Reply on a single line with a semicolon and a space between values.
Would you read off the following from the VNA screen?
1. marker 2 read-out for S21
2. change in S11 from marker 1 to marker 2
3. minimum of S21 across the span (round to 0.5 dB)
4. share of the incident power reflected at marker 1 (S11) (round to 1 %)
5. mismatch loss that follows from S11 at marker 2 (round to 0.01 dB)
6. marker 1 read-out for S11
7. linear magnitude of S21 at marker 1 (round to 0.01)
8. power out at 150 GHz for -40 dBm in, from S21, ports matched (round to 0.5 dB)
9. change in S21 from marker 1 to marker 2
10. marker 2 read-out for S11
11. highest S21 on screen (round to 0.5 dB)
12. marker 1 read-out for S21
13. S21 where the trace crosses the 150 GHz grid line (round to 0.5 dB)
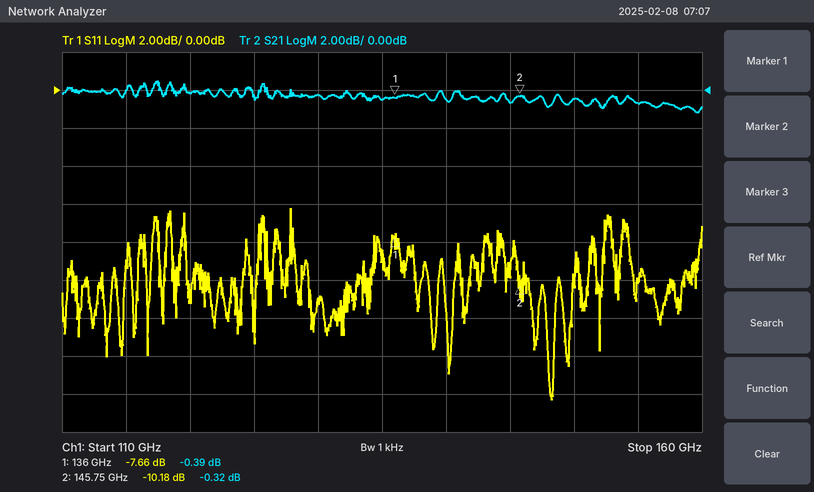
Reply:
-0.32 dB; -2.52 dB; -1.0 dB; 17 %; 0.44 dB; -7.66 dB; 0.96; -40.5 dBm; 0.07 dB; -10.18 dB; 0.5 dB; -0.39 dB; -0.5 dB
